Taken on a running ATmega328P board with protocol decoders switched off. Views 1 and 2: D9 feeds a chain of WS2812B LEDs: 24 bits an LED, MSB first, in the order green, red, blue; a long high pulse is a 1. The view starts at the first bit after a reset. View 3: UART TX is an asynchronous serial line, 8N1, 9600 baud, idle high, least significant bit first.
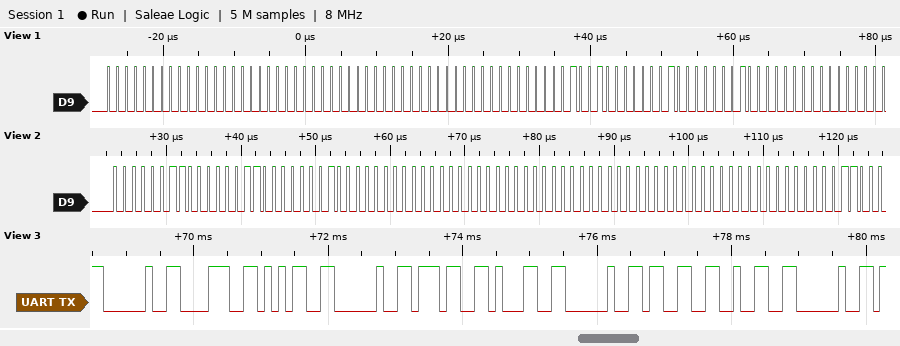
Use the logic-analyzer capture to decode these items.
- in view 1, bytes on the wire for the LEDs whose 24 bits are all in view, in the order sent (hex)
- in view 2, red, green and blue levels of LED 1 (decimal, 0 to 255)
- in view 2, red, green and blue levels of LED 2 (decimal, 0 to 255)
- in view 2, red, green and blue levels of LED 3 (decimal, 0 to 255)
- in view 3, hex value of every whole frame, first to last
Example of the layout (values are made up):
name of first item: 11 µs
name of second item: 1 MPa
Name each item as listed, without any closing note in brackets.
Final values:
in view 1, bytes on the wire for the LEDs whose 24 bits are all in view, in the order sent: 00 00 00 00 00 00 09 01 01
in view 2, red, green and blue levels of LED 1: 3, 3, 1
in view 2, red, green and blue levels of LED 2: 0, 0, 0
in view 2, red, green and blue levels of LED 3: 0, 0, 0
in view 3, hex value of every whole frame, first to last: 0x20 0x38 0x35 0x20 0x37 0x31 0x20 0x33 0x32 0x20
